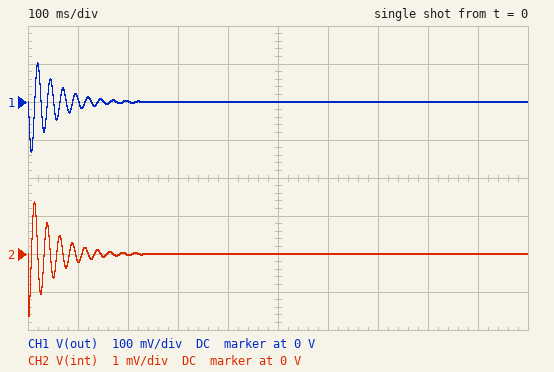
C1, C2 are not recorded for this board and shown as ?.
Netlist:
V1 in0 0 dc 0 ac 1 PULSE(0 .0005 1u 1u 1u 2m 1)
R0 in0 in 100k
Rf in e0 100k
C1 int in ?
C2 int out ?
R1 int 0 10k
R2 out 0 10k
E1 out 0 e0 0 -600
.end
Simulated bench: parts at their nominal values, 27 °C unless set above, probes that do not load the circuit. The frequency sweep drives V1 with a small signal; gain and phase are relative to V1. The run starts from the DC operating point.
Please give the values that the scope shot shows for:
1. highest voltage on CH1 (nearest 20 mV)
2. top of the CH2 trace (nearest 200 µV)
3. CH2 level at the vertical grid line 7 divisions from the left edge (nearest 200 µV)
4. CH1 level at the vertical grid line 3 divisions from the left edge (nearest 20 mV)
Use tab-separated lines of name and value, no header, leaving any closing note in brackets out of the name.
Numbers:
highest voltage on CH1	100 mV
top of the CH2 trace	1.4 mV
CH2 level at the vertical grid line 7 divisions from the left edge	0 V
CH1 level at the vertical grid line 3 divisions from the left edge	0 V
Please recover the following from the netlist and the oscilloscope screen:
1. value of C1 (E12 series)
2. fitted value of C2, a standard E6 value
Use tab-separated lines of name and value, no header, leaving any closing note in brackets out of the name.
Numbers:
value of C1	5.6 nF
fitted value of C2, a standard E6 value	4.7 nF
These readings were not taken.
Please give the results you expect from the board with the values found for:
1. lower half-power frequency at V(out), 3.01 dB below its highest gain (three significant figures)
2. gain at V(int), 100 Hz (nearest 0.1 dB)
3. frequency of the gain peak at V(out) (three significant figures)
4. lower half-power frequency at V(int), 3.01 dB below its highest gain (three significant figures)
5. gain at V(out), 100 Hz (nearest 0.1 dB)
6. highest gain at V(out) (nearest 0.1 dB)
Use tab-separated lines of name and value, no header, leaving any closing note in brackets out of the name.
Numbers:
lower half-power frequency at V(out), 3.01 dB below its highest gain	36.2 Hz
gain at V(int), 100 Hz	10.5 dB
frequency of the gain peak at V(out)	39.7 Hz
lower half-power frequency at V(int), 3.01 dB below its highest gain	36.8 Hz
gain at V(out), 100 Hz	41.2 dB
highest gain at V(out)	71.2 dB
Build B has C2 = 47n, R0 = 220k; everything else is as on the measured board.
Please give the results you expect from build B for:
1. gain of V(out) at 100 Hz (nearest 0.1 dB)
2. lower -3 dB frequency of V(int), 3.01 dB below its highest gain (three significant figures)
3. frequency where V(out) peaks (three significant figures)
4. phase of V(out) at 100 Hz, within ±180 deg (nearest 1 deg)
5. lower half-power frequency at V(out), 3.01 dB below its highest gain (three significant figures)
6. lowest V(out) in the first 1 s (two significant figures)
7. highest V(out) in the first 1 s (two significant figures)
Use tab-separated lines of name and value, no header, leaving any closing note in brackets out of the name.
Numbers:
gain of V(out) at 100 Hz	13.3 dB
lower -3 dB frequency of V(int), 3.01 dB below its highest gain	8.14 Hz
frequency where V(out) peaks	8.51 Hz
phase of V(out) at 100 Hz, within ±180 deg	19 deg
lower half-power frequency at V(out), 3.01 dB below its highest gain	8.10 Hz
lowest V(out) in the first 1 s	-30 mV
highest V(out) in the first 1 s	26 mV
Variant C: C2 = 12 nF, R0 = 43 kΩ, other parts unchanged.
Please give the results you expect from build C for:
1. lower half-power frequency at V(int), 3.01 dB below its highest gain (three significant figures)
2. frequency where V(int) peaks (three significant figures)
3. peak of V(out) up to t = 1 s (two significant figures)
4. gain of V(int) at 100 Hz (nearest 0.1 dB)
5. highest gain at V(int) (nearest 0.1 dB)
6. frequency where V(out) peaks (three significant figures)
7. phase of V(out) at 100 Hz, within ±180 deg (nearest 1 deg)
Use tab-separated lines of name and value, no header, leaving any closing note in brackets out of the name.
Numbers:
lower half-power frequency at V(int), 3.01 dB below its highest gain	36.3 Hz
frequency where V(int) peaks	38.2 Hz
peak of V(out) up to t = 1 s	110 mV
gain of V(int) at 100 Hz	17.7 dB
highest gain at V(int)	44.7 dB
frequency where V(out) peaks	38.1 Hz
phase of V(out) at 100 Hz, within ±180 deg	9 deg
